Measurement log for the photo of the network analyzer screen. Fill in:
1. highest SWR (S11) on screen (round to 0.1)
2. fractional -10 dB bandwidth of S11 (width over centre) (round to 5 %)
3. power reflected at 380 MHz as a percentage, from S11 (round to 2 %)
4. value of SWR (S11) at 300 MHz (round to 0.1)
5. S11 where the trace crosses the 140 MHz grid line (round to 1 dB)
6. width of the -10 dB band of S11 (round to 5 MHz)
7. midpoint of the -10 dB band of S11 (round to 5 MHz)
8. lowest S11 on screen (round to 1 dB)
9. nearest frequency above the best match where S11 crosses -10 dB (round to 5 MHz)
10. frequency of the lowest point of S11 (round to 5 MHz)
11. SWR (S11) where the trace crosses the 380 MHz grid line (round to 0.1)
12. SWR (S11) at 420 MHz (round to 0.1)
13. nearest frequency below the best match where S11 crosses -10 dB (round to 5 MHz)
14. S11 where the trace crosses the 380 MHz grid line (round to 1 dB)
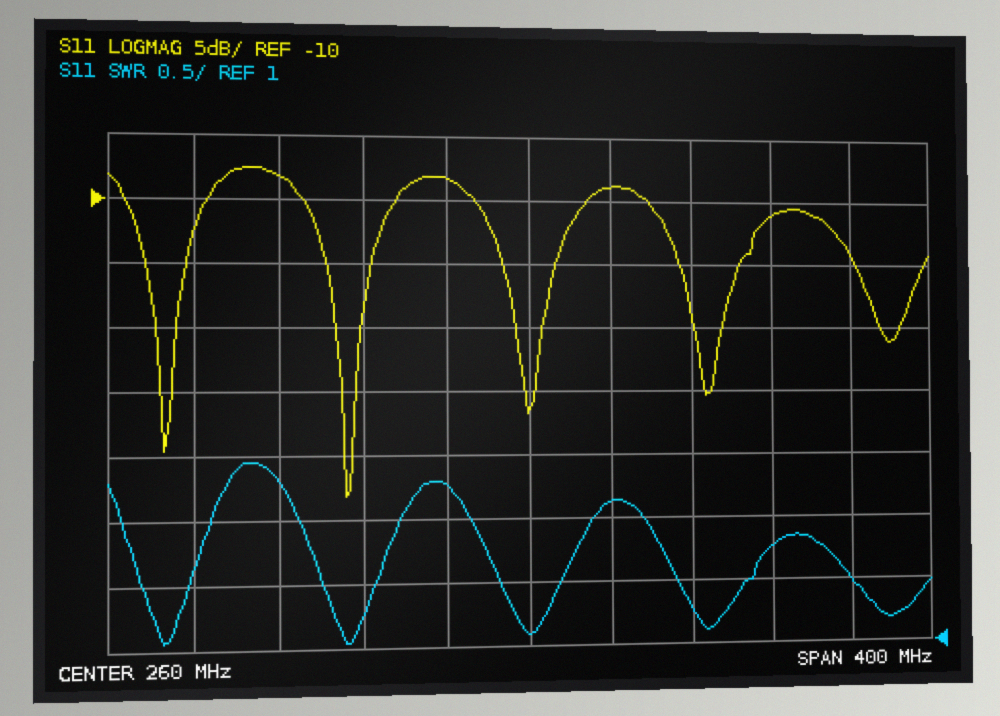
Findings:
2.5
25 %
8 %
2.1
-8 dB
45 MHz
175 MHz
-33 dB
195 MHz
170 MHz
1.8
1.5
150 MHz
-11 dB
